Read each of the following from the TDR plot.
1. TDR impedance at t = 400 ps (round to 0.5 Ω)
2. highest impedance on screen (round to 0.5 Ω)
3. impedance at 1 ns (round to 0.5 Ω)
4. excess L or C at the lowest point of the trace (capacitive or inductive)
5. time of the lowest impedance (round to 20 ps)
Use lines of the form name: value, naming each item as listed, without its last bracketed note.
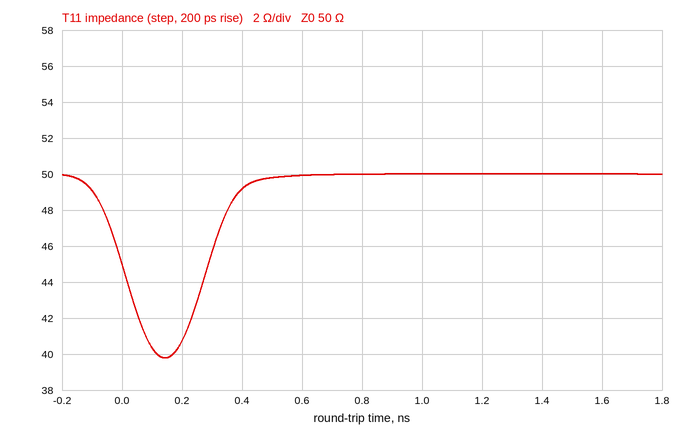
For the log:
TDR impedance at t = 400 ps: 49.0 Ω
highest impedance on screen: 50.0 Ω
impedance at 1 ns: 50.0 Ω
excess L or C at the lowest point of the trace: capacitive
time of the lowest impedance: 140 ps
